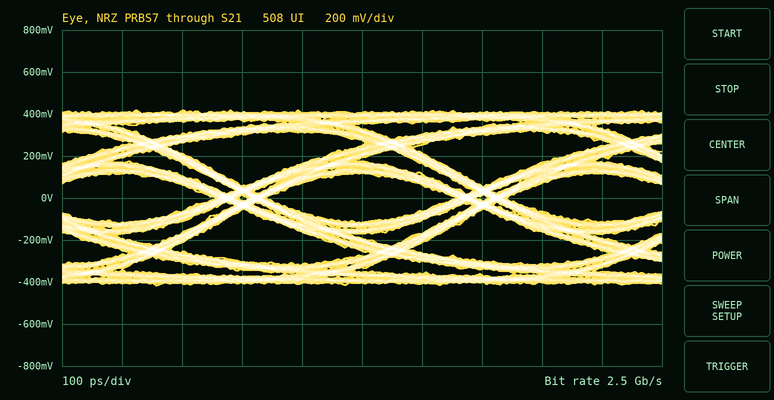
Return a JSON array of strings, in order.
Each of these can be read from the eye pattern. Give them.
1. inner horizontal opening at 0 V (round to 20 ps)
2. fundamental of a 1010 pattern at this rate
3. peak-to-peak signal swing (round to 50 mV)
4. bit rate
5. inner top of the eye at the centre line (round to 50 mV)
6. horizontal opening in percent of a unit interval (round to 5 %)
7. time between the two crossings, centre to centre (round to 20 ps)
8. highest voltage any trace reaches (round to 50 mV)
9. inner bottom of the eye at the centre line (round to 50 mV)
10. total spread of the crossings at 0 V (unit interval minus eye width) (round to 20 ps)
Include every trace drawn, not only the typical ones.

["320 ps", "1.25 GHz", "850 mV", "2.5 Gb/s", "100 mV", "80 %", "400 ps", "400 mV", "-100 mV", "80 ps"]
